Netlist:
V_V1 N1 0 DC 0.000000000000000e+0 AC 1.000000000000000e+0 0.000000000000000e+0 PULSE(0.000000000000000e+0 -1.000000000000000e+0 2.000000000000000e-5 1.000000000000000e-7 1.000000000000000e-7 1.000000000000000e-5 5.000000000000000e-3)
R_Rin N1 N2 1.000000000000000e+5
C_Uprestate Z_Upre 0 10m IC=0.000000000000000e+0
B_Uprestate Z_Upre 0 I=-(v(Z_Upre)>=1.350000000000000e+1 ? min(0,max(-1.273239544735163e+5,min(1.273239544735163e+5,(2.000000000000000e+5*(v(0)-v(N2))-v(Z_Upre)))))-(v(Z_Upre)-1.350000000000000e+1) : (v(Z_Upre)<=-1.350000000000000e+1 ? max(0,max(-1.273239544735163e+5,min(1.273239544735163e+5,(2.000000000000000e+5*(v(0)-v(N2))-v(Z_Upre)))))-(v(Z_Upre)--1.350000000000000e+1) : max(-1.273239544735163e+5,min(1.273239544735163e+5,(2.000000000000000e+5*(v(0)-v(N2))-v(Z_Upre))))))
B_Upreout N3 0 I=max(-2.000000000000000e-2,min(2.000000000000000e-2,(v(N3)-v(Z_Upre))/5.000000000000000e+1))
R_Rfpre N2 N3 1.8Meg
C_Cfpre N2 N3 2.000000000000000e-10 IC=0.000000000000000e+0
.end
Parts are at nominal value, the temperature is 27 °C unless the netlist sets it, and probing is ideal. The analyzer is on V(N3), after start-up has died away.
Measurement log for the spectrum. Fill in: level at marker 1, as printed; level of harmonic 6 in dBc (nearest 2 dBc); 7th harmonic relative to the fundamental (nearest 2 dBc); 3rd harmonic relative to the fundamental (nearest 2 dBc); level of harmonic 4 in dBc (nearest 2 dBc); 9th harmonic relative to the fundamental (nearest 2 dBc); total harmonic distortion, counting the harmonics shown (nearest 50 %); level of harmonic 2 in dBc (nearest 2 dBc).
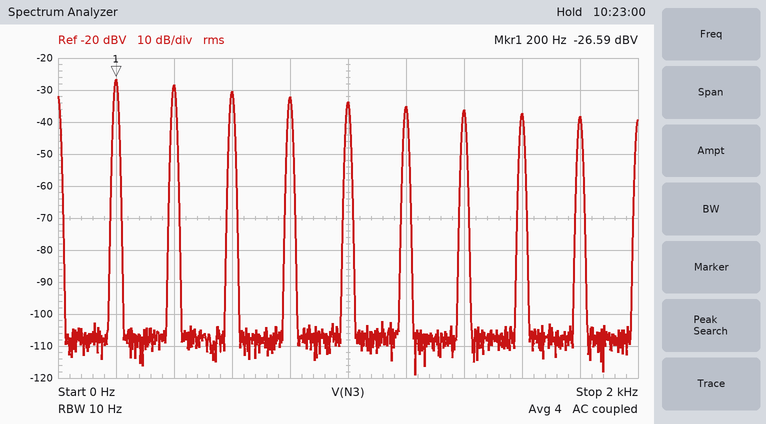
-26.59 dBV
-8 dBc
-10 dBc
-4 dBc
-6 dBc
-12 dBc
150 %
-2 dBc
